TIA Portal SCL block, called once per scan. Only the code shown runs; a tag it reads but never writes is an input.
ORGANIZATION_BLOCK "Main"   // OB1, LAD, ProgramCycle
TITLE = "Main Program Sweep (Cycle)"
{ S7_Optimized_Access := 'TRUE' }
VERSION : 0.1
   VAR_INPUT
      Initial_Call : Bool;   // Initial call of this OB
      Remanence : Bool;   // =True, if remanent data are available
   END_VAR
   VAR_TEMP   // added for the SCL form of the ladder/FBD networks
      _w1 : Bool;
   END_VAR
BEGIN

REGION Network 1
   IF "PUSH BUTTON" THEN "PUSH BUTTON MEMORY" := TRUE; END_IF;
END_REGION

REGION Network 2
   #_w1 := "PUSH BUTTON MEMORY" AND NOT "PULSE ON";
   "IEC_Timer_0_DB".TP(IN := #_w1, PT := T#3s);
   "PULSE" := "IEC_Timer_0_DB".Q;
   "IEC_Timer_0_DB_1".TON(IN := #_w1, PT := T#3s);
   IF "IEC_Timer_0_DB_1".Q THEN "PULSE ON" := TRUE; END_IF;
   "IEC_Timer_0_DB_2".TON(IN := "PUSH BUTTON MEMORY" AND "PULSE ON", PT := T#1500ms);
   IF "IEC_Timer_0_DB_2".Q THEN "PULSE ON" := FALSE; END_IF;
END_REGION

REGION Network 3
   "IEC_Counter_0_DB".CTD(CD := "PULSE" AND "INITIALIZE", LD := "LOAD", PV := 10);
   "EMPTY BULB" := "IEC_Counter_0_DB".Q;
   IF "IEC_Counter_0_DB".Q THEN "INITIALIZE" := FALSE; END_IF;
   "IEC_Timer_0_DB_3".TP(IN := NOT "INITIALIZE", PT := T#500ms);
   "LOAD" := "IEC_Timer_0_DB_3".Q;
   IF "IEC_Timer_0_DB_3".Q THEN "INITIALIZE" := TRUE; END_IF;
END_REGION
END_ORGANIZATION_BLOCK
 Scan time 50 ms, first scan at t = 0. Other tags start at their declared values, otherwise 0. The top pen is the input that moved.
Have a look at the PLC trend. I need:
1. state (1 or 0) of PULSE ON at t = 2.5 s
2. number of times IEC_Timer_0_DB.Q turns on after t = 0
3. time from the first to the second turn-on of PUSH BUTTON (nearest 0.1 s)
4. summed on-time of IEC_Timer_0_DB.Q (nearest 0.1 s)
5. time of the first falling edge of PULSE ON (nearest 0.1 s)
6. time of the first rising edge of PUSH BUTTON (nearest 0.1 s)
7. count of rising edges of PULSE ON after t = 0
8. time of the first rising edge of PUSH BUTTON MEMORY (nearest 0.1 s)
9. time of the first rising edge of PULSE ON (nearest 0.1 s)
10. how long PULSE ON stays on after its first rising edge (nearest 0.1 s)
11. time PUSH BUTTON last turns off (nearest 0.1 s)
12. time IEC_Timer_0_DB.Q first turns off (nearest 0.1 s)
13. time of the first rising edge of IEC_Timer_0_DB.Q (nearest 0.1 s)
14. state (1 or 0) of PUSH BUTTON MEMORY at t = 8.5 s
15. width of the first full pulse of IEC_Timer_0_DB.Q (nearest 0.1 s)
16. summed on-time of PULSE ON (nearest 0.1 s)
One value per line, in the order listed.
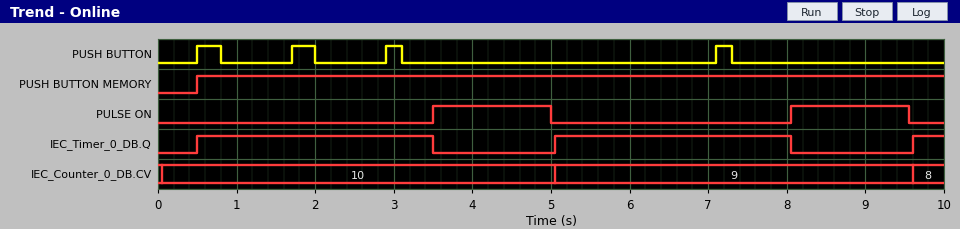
0
3
1.2 s
6.4 s
5.0 s
0.5 s
2
0.5 s
3.5 s
1.5 s
7.3 s
3.5 s
0.5 s
1
3.0 s
3.0 s
